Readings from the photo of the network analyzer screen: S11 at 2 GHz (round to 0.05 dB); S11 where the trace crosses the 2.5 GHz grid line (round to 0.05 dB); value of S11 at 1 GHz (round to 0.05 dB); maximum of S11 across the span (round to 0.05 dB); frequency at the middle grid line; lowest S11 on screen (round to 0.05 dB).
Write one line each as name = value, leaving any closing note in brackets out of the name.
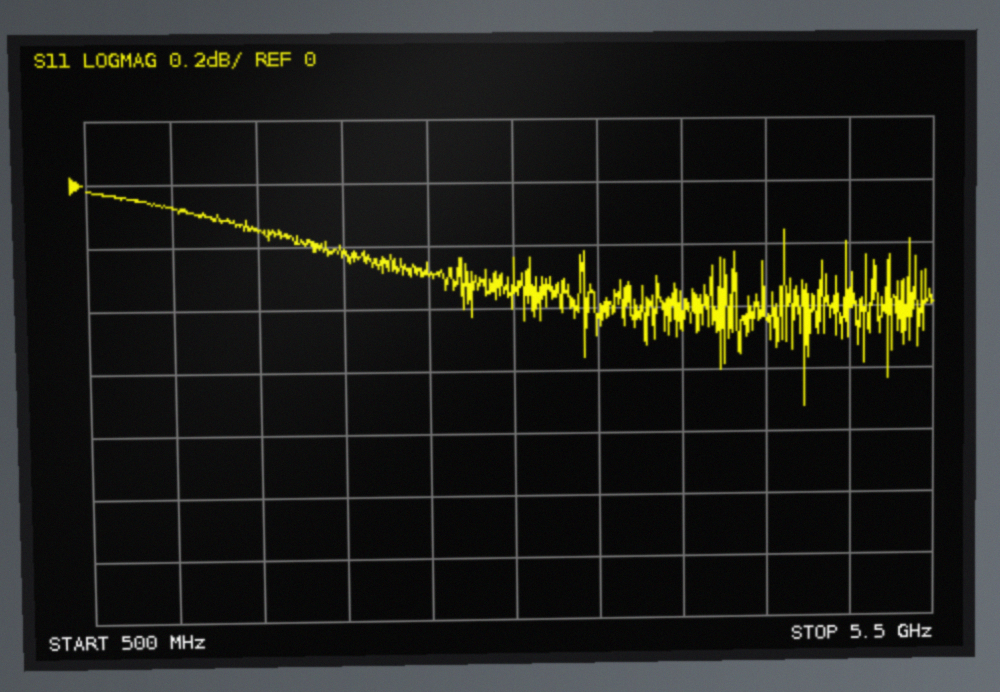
S11 at 2 GHz = -0.20 dB
S11 where the trace crosses the 2.5 GHz grid line = -0.30 dB
value of S11 at 1 GHz = -0.05 dB
maximum of S11 across the span = 0.00 dB
frequency at the middle grid line = 3 GHz
lowest S11 on screen = -0.70 dB
